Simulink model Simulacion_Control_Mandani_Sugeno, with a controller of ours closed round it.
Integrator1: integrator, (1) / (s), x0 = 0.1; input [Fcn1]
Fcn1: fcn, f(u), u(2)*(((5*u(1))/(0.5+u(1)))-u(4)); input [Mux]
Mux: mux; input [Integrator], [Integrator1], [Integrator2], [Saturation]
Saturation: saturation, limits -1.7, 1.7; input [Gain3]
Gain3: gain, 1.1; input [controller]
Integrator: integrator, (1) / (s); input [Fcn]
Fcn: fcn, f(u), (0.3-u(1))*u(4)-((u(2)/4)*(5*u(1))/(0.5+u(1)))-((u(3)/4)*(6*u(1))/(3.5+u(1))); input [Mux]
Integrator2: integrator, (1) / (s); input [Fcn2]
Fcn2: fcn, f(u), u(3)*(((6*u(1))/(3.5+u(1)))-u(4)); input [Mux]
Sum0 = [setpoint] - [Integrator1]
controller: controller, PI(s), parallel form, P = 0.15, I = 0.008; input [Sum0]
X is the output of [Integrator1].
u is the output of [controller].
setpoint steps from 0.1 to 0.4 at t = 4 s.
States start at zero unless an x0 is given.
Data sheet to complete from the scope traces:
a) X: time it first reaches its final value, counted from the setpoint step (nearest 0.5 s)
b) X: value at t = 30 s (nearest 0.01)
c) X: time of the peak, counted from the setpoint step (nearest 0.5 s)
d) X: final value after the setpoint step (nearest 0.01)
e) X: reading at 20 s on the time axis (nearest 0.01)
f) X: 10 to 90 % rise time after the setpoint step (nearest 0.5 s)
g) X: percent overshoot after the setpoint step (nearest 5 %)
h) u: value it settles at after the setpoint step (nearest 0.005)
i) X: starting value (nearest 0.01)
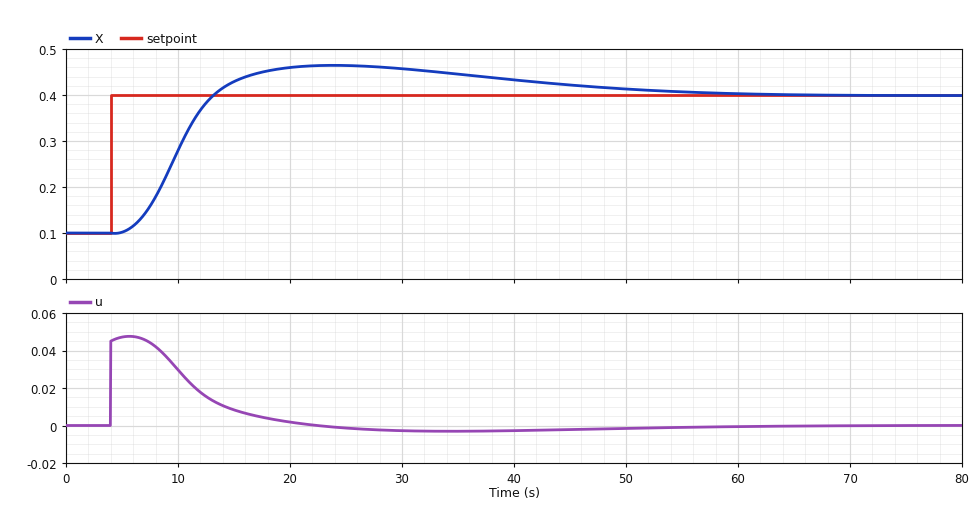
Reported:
9.0 s
0.46
20.0 s
0.40
0.46
5.5 s
20 %
0.000
0.10
